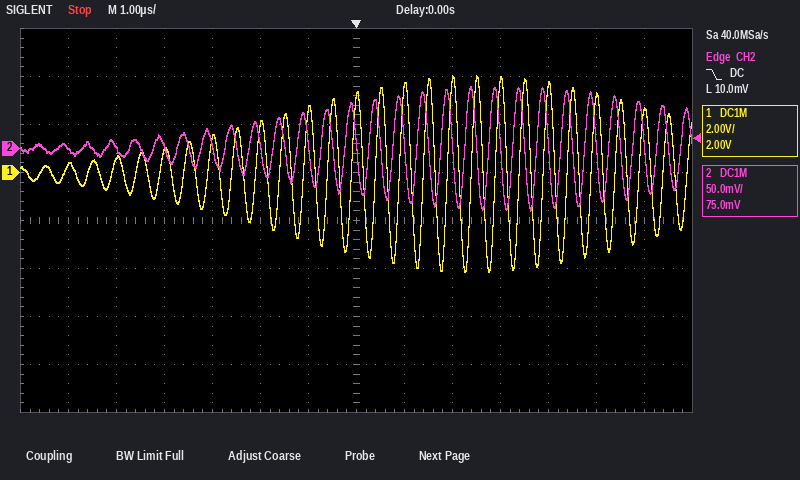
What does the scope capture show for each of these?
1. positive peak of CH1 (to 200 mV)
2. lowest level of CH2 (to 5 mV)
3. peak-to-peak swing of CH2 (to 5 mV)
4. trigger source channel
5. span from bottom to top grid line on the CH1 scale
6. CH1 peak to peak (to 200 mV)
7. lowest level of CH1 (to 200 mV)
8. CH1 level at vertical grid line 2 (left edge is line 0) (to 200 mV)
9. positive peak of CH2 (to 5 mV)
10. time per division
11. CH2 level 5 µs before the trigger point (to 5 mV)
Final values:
4.0 V
-65 mV
130 mV
CH2
16 V
8.2 V
-4.2 V
600 mV
65 mV
1 µs
0 mV
